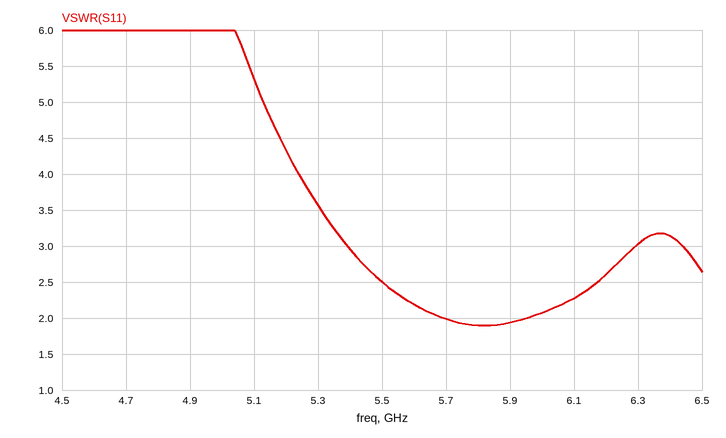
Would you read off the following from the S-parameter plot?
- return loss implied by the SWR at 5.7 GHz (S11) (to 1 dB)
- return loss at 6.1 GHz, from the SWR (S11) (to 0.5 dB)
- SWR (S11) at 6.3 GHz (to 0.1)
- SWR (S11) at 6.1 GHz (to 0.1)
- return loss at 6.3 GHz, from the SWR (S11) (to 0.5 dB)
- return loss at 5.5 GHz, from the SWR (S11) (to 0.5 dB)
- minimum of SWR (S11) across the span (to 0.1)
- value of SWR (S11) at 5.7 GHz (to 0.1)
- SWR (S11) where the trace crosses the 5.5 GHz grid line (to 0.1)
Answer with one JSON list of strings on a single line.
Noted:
["10 dB", "8.0 dB", "3.0", "2.3", "6.0 dB", "7.5 dB", "1.9", "2.0", "2.5"]
